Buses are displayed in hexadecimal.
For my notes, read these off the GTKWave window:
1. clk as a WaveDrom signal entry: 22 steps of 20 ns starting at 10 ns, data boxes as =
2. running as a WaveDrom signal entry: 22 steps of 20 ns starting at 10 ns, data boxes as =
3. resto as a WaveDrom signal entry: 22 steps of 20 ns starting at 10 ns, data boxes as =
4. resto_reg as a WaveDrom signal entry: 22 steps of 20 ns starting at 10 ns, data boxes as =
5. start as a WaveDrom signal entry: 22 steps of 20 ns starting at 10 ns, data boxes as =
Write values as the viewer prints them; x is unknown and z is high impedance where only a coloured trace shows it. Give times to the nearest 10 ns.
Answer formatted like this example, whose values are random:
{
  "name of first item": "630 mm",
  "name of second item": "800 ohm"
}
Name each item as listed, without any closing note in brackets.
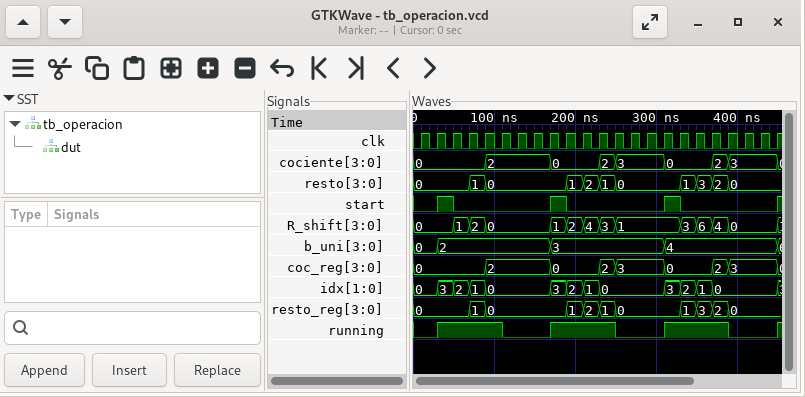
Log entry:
{
  "clk as a WaveDrom signal entry: 22 steps of 20 ns starting at 10 ns, data boxes as =": "{name: 'clk', wave: 'p.....................'}",
  "running as a WaveDrom signal entry: 22 steps of 20 ns starting at 10 ns, data boxes as =": "{name: 'running', wave: '01...0..1...0..1...0..'}",
  "resto as a WaveDrom signal entry: 22 steps of 20 ns starting at 10 ns, data boxes as =": "{name: 'resto', wave: '=..==....====...====..', data: '0 1 0 1 2 1 0 1 3 2 0'}",
  "resto_reg as a WaveDrom signal entry: 22 steps of 20 ns starting at 10 ns, data boxes as =": "{name: 'resto_reg', wave: '=..==....====...====..', data: '0 1 0 1 2 1 0 1 3 2 0'}",
  "start as a WaveDrom signal entry: 22 steps of 20 ns starting at 10 ns, data boxes as =": "{name: 'start', wave: '010.....10.....10.....'}"
}
